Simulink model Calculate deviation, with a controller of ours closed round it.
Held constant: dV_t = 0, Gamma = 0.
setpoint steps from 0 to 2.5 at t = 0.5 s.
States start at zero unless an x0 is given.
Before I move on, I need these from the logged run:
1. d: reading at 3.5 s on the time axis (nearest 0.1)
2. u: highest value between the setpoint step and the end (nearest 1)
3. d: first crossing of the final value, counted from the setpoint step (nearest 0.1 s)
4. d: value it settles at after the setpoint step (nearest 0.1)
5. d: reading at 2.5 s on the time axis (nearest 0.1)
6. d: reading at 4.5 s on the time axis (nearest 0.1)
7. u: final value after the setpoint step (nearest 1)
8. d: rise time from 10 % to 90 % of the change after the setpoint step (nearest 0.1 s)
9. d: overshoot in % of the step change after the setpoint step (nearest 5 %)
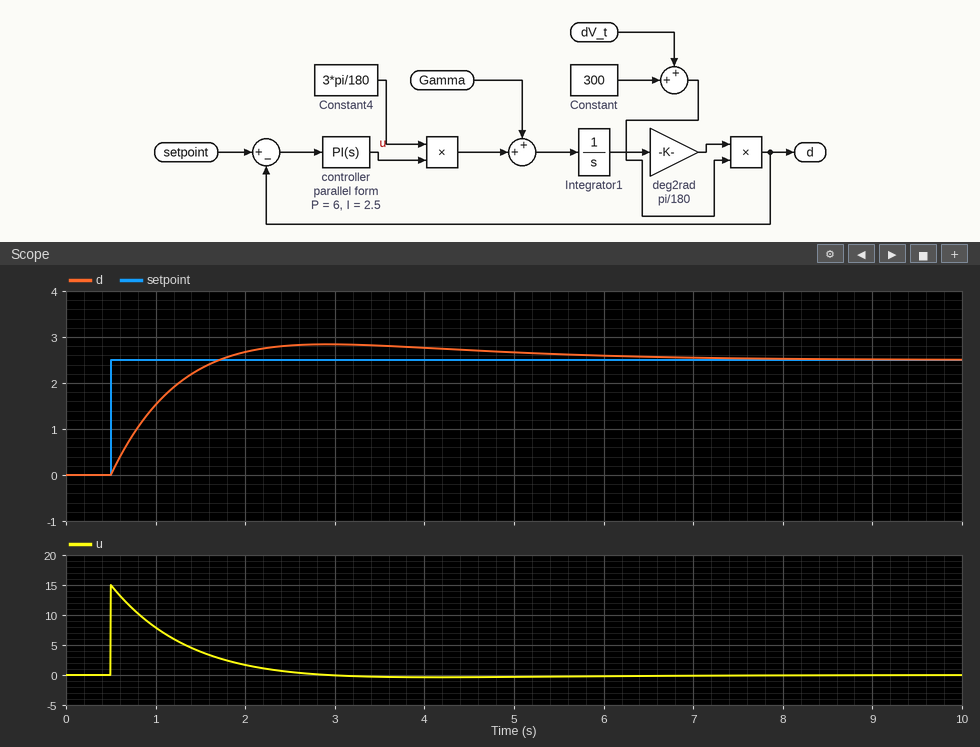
2.8
15
1.2 s
2.5
2.8
2.7
0
0.9 s
15 %
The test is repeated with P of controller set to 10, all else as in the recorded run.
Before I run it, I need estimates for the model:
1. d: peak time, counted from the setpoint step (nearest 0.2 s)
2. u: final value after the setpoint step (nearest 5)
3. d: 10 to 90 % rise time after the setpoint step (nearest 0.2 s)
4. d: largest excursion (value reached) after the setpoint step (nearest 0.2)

2.0 s
0
0.6 s
2.6
